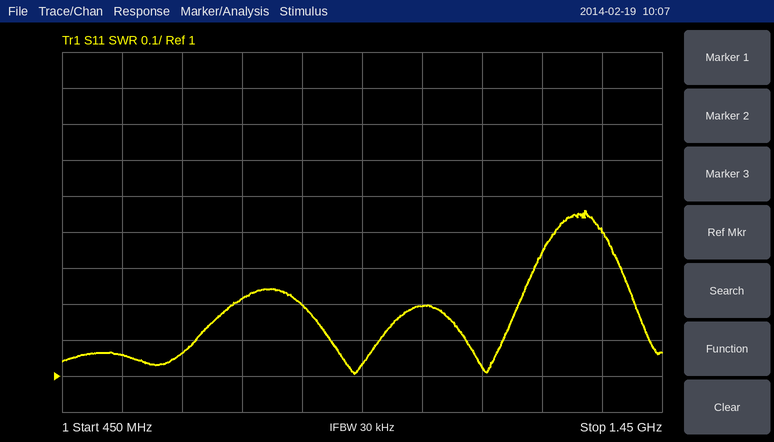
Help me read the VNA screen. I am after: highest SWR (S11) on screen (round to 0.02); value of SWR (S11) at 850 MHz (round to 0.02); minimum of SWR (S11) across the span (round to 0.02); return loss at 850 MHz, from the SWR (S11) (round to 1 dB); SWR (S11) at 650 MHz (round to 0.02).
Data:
1.46
1.20
1.00
21 dB
1.06
